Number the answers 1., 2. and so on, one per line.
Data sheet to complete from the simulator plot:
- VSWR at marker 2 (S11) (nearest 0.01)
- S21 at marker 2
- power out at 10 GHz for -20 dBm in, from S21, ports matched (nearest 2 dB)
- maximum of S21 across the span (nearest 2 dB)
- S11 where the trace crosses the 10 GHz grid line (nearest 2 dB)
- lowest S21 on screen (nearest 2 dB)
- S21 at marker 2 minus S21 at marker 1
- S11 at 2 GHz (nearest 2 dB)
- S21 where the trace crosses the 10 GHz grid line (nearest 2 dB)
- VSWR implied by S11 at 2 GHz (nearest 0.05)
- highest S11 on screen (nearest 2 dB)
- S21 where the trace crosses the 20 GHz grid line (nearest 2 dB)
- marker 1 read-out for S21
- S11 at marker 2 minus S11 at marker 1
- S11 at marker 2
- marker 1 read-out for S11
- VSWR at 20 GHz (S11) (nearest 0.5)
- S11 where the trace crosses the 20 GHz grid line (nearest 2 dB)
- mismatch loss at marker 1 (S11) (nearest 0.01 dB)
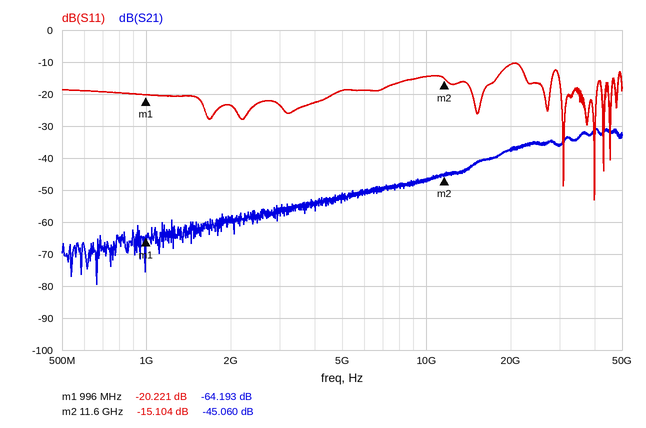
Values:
1. 1.43
2. -45.060 dB
3. -66 dBm
4. -30 dB
5. -14 dB
6. -80 dB
7. 19.133 dB
8. -24 dB
9. -46 dB
10. 1.15
11. -10 dB
12. -38 dB
13. -64.193 dB
14. 5.117 dB
15. -15.104 dB
16. -20.221 dB
17. 2.0
18. -10 dB
19. 0.04 dB
